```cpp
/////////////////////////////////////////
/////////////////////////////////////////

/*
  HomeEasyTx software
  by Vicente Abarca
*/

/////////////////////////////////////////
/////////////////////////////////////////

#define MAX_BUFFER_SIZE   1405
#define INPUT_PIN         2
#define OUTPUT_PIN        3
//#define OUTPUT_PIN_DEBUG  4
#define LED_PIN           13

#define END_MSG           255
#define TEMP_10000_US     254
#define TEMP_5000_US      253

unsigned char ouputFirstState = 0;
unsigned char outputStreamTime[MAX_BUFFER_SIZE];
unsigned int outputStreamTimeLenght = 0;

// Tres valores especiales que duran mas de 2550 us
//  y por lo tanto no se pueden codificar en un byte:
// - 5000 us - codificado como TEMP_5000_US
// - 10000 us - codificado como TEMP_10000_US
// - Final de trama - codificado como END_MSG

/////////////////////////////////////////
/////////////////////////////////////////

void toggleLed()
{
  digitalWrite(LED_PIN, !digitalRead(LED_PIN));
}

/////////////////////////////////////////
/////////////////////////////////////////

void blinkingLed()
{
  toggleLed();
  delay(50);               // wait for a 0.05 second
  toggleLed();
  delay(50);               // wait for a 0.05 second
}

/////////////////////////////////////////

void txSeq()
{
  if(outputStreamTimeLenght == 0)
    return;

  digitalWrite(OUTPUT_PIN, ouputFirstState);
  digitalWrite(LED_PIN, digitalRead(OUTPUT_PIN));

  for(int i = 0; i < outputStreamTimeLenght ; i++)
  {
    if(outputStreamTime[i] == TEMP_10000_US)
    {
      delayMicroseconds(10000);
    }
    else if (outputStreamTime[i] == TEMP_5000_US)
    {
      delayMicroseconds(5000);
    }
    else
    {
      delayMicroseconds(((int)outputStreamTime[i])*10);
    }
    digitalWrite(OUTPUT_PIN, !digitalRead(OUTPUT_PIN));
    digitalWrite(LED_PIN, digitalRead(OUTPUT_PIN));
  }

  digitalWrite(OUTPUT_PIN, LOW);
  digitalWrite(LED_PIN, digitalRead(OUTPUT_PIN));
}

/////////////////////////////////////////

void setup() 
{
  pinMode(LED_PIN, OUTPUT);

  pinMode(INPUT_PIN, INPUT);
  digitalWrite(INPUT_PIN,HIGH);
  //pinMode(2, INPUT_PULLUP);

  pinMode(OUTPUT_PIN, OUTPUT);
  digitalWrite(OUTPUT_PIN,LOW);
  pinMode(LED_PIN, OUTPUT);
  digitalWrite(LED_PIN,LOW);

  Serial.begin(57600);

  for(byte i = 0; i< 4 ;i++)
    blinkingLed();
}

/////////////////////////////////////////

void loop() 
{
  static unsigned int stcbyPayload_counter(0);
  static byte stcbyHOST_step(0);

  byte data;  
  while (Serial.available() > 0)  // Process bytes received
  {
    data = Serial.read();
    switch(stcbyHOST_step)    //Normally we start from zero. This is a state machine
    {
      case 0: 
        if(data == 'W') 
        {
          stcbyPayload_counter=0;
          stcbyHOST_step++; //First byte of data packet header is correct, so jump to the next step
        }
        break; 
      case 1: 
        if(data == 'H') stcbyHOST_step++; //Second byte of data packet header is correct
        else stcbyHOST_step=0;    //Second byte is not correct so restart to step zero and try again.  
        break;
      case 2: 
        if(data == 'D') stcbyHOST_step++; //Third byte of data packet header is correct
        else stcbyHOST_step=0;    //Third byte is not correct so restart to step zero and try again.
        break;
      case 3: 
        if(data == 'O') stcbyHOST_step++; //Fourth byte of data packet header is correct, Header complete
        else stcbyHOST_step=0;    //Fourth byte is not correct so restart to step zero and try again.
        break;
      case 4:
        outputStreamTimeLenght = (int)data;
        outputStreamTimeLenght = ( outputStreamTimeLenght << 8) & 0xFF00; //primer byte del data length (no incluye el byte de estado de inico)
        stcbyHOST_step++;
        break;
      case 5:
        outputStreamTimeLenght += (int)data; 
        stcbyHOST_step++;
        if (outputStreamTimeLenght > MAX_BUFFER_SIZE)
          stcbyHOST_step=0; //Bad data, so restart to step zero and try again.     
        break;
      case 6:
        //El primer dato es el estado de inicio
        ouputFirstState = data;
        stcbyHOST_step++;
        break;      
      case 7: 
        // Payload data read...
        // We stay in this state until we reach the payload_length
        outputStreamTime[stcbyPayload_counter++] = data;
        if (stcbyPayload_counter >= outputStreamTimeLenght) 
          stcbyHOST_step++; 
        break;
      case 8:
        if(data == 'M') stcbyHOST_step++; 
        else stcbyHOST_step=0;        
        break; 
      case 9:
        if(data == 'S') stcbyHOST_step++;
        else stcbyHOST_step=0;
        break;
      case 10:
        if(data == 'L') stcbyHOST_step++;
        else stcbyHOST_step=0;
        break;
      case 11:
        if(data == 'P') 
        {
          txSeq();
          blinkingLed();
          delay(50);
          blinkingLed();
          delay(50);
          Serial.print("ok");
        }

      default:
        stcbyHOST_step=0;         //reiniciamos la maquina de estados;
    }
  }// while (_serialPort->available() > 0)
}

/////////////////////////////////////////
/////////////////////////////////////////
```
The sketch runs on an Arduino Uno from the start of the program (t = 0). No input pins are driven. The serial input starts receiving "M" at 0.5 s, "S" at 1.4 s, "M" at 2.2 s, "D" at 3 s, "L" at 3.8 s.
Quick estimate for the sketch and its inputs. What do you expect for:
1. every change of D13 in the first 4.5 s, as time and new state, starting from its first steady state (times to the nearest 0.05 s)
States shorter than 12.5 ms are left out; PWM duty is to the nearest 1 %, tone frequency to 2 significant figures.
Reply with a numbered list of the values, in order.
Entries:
1. 0 s high; 0.05 s low; 0.1 s high; 0.15 s low; 0.2 s high; 0.25 s low; 0.3 s high; 0.35 s low
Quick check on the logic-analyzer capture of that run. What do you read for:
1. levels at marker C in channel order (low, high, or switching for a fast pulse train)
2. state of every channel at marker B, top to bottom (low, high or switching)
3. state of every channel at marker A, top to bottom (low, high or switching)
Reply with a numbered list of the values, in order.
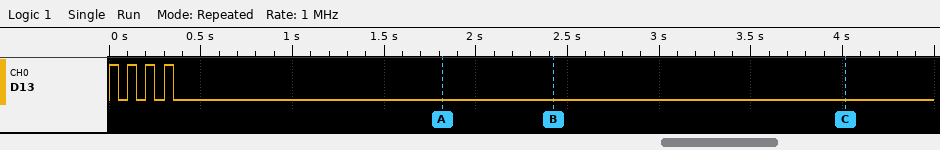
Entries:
1. D13 low
2. D13 low
3. D13 low
